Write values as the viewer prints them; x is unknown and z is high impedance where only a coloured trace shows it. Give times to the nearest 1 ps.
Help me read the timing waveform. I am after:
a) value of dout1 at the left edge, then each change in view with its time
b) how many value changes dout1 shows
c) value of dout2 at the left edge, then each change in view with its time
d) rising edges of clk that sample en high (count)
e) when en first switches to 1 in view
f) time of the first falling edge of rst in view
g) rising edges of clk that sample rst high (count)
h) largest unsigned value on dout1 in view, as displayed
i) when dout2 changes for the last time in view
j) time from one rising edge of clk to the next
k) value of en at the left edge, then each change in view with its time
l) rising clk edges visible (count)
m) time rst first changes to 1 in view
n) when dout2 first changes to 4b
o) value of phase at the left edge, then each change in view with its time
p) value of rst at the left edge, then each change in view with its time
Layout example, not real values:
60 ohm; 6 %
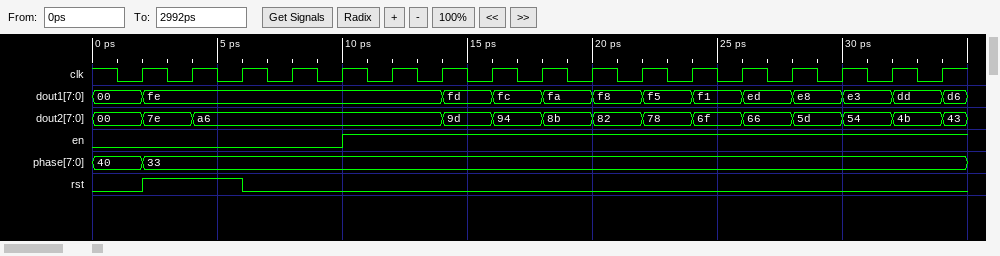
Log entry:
00, fe at 2 ps, fd at 14 ps, fc at 16 ps, fa at 18 ps, f8 at 20 ps, f5 at 22 ps, f1 at 24 ps, ed at 26 ps, e8 at 28 ps, e3 at 30 ps, dd at 32 ps, d6 at 34 ps; 12; 00, 7e at 2 ps, a6 at 4 ps, 9d at 14 ps, 94 at 16 ps, 8b at 18 ps, 82 at 20 ps, 78 at 22 ps, 6f at 24 ps, 66 at 26 ps, 5d at 28 ps, 54 at 30 ps, 4b at 32 ps, 43 at 34 ps; 12; 10 ps; 6 ps; 2; fe; 34 ps; 2 ps; 0, 1 at 10 ps; 17; 2 ps; 32 ps; 40, 33 at 2 ps; 0, 1 at 2 ps, 0 at 6 ps
